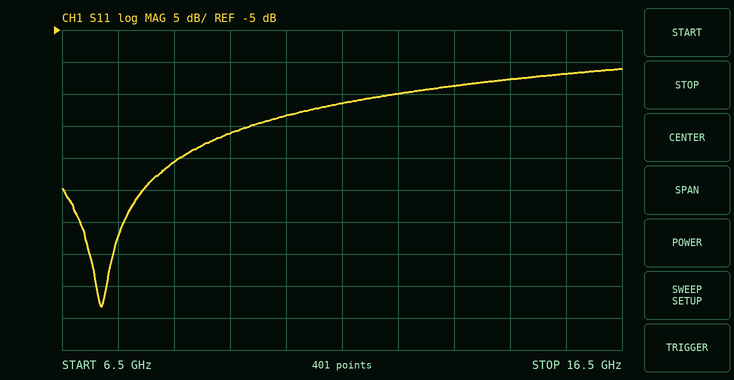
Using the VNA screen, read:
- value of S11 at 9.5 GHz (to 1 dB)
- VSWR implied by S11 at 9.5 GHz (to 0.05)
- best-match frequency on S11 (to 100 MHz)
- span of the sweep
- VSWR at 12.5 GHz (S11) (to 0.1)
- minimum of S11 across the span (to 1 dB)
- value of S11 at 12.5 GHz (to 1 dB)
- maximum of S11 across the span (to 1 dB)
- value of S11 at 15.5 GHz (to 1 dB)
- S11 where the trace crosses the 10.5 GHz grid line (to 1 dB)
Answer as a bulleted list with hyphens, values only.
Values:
- -21 dB
- 1.20
- 7.2 GHz
- 10 GHz
- 1.4
- -48 dB
- -15 dB
- -11 dB
- -12 dB
- -18 dB
